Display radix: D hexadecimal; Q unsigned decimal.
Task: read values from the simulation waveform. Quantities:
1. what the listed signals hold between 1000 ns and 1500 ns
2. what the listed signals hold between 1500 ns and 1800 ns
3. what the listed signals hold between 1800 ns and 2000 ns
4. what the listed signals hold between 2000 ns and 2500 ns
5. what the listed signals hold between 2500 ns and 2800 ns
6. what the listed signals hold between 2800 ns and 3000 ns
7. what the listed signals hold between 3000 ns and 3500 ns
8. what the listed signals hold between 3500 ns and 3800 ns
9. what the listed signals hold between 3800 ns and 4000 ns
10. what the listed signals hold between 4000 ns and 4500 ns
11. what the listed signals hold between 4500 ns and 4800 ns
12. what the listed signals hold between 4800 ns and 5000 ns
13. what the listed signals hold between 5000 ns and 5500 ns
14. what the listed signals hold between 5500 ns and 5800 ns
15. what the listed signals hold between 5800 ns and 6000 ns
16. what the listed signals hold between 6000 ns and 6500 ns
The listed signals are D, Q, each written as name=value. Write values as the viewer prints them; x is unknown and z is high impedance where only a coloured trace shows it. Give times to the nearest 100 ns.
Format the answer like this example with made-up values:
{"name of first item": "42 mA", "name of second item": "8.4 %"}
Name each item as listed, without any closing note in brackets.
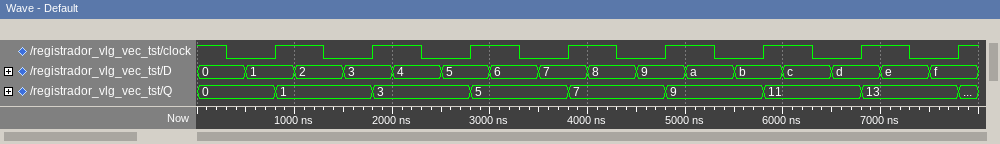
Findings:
{"what the listed signals hold between 1000 ns and 1500 ns": "D=2, Q=1", "what the listed signals hold between 1500 ns and 1800 ns": "D=3, Q=1", "what the listed signals hold between 1800 ns and 2000 ns": "D=3, Q=3", "what the listed signals hold between 2000 ns and 2500 ns": "D=4, Q=3", "what the listed signals hold between 2500 ns and 2800 ns": "D=5, Q=3", "what the listed signals hold between 2800 ns and 3000 ns": "D=5, Q=5", "what the listed signals hold between 3000 ns and 3500 ns": "D=6, Q=5", "what the listed signals hold between 3500 ns and 3800 ns": "D=7, Q=5", "what the listed signals hold between 3800 ns and 4000 ns": "D=7, Q=7", "what the listed signals hold between 4000 ns and 4500 ns": "D=8, Q=7", "what the listed signals hold between 4500 ns and 4800 ns": "D=9, Q=7", "what the listed signals hold between 4800 ns and 5000 ns": "D=9, Q=9", "what the listed signals hold between 5000 ns and 5500 ns": "D=a, Q=9", "what the listed signals hold between 5500 ns and 5800 ns": "D=b, Q=9", "what the listed signals hold between 5800 ns and 6000 ns": "D=b, Q=11", "what the listed signals hold between 6000 ns and 6500 ns": "D=c, Q=11"}
